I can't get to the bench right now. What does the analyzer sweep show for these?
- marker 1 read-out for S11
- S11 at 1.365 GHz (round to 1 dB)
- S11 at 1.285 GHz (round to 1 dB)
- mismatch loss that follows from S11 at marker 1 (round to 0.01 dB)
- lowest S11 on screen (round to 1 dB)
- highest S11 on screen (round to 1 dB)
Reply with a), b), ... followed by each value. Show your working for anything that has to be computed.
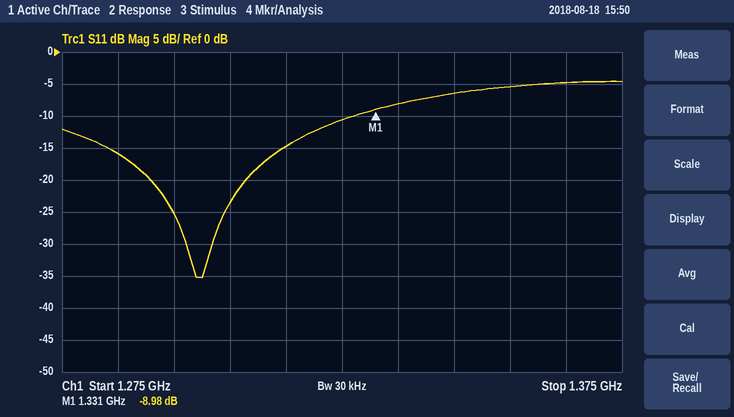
a) -8.98 dB
b) -5 dB
c) -16 dB
d) −10 log10(1 − 10^(-8.98/10)) ≈ 0.59 dB
e) -35 dB
f) -5 dB
